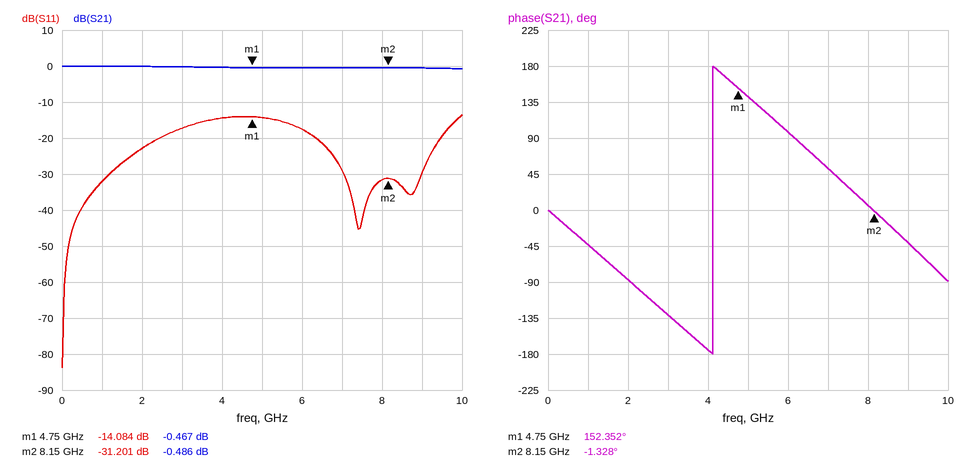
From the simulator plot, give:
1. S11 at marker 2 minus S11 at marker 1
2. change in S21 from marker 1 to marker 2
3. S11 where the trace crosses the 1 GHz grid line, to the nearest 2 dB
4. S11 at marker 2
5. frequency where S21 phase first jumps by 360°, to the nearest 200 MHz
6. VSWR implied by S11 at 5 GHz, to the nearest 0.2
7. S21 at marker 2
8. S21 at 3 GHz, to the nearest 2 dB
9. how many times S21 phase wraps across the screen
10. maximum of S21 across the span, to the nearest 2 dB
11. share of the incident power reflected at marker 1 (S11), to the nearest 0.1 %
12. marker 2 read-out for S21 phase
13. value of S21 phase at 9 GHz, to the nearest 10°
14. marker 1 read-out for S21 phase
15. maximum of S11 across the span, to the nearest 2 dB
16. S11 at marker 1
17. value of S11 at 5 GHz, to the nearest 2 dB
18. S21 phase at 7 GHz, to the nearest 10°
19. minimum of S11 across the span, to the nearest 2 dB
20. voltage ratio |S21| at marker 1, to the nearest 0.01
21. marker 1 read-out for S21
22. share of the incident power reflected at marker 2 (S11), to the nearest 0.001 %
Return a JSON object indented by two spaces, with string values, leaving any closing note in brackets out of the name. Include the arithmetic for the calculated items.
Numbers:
{
  "S11 at marker 2 minus S11 at marker 1": "-31.201 − (-14.084) = -17.117 dB",
  "change in S21 from marker 1 to marker 2": "-0.486 − (-0.467) = -0.019 dB",
  "S11 where the trace crosses the 1 GHz grid line, to the nearest 2 dB": "-32 dB",
  "S11 at marker 2": "-31.201 dB",
  "frequency where S21 phase first jumps by 360°, to the nearest 200 MHz": "4.2 GHz",
  "VSWR implied by S11 at 5 GHz, to the nearest 0.2": "|Γ| = 10^(-14/20) = 0.1995; VSWR = (1 + 0.1995)/(1 − 0.1995) ≈ 1.50, so 1.4 to the nearest 0.2",
  "S21 at marker 2": "-0.486 dB",
  "S21 at 3 GHz, to the nearest 2 dB": "0 dB",
  "how many times S21 phase wraps across the screen": "1",
  "maximum of S21 across the span, to the nearest 2 dB": "0 dB",
  "share of the incident power reflected at marker 1 (S11), to the nearest 0.1 %": "10^(-14.084/10) ≈ 3.9 %",
  "marker 2 read-out for S21 phase": "-1.328°",
  "value of S21 phase at 9 GHz, to the nearest 10°": "-40°",
  "marker 1 read-out for S21 phase": "152.352°",
  "maximum of S11 across the span, to the nearest 2 dB": "-14 dB",
  "S11 at marker 1": "-14.084 dB",
  "value of S11 at 5 GHz, to the nearest 2 dB": "-14 dB",
  "S21 phase at 7 GHz, to the nearest 10°": "50°",
  "minimum of S11 across the span, to the nearest 2 dB": "-84 dB",
  "voltage ratio |S21| at marker 1, to the nearest 0.01": "10^(-0.467/20) ≈ 0.95",
  "marker 1 read-out for S21": "-0.467 dB",
  "share of the incident power reflected at marker 2 (S11), to the nearest 0.001 %": "10^(-31.201/10) ≈ 0.076 %"
}
